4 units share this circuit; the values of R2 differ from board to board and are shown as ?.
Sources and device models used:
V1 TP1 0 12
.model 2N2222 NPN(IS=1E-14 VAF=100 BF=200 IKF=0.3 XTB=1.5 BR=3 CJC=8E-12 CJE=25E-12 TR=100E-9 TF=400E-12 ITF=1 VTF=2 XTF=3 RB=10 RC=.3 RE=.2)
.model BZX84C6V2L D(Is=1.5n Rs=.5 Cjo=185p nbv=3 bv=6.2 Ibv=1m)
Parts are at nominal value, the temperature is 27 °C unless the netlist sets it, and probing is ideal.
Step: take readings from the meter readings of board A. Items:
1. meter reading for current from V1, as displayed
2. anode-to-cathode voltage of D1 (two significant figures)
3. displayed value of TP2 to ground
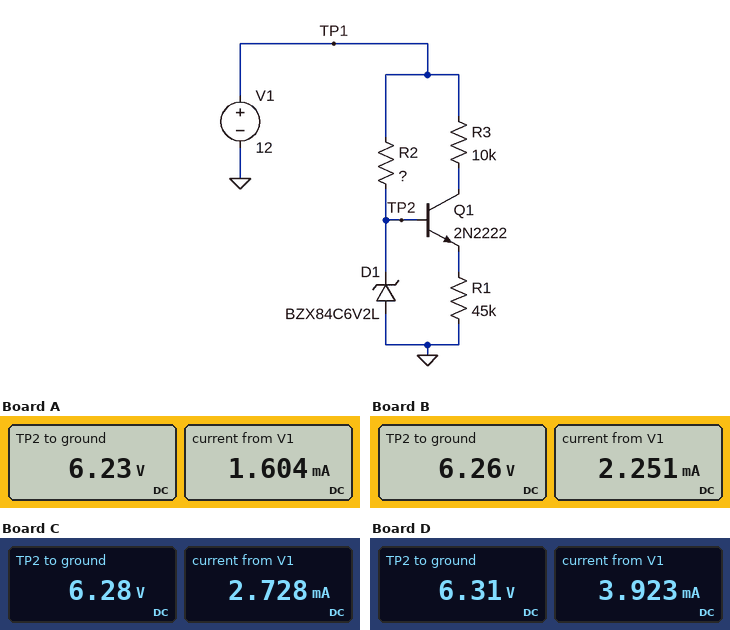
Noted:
1.604 mA
-6.2 V
6.23 V
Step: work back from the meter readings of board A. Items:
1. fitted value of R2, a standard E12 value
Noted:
3.9 kΩ
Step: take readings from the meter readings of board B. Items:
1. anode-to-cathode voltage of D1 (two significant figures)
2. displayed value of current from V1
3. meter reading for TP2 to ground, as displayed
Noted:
-6.3 V
2.251 mA
6.26 V
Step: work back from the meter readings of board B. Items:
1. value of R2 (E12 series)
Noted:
2.7 kΩ
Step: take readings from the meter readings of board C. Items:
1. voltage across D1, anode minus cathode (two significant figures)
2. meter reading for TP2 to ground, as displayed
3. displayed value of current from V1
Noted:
-6.3 V
6.28 V
2.728 mA
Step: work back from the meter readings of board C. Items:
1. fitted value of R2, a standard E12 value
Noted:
2.2 kΩ
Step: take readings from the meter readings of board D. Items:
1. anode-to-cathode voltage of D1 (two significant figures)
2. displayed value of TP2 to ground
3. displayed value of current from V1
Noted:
-6.3 V
6.31 V
3.923 mA
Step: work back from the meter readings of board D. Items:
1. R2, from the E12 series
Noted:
1.5 kΩ
